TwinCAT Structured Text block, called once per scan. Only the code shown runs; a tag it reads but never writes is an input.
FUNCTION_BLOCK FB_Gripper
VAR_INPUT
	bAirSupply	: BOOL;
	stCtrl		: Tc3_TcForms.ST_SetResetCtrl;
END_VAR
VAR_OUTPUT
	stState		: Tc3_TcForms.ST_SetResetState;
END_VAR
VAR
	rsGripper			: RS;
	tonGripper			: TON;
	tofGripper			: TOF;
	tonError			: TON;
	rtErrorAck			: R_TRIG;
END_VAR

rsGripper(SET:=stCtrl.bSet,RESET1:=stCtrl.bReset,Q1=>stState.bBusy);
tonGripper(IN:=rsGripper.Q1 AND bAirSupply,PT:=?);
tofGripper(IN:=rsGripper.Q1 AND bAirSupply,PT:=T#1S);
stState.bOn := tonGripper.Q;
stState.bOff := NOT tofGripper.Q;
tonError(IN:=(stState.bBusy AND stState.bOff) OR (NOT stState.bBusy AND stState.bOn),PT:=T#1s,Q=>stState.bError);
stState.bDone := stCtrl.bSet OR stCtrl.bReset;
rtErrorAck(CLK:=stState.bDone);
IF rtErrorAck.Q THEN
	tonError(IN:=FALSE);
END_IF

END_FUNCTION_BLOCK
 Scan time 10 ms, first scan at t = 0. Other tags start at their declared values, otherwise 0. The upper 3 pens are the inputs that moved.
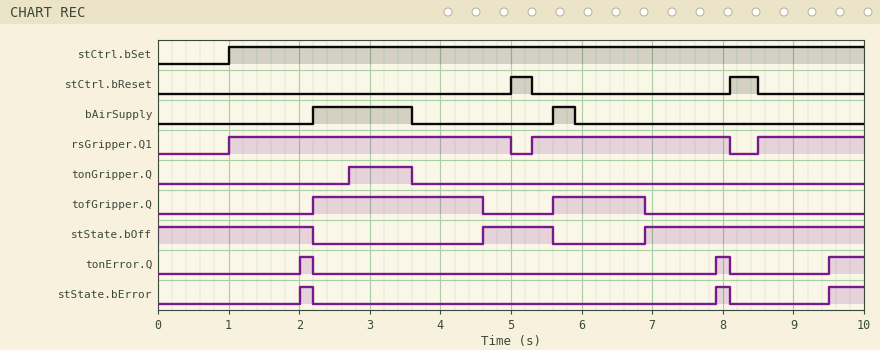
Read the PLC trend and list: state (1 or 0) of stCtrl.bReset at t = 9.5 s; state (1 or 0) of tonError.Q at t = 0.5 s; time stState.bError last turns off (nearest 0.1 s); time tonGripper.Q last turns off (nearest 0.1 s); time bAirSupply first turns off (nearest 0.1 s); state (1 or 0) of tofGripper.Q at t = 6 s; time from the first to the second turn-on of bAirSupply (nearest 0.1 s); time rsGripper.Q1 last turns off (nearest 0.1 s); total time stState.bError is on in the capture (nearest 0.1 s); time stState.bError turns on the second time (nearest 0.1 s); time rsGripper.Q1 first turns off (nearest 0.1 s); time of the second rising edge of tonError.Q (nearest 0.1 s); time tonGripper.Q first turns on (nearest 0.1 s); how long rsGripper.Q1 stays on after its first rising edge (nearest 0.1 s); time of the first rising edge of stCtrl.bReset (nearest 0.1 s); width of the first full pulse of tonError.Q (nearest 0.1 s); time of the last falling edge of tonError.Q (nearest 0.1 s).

0
0
8.1 s
3.6 s
3.6 s
1
3.4 s
8.1 s
0.9 s
7.9 s
5.0 s
7.9 s
2.7 s
4.0 s
5.0 s
0.2 s
8.1 s
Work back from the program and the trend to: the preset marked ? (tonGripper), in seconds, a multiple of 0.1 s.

0.5 s
